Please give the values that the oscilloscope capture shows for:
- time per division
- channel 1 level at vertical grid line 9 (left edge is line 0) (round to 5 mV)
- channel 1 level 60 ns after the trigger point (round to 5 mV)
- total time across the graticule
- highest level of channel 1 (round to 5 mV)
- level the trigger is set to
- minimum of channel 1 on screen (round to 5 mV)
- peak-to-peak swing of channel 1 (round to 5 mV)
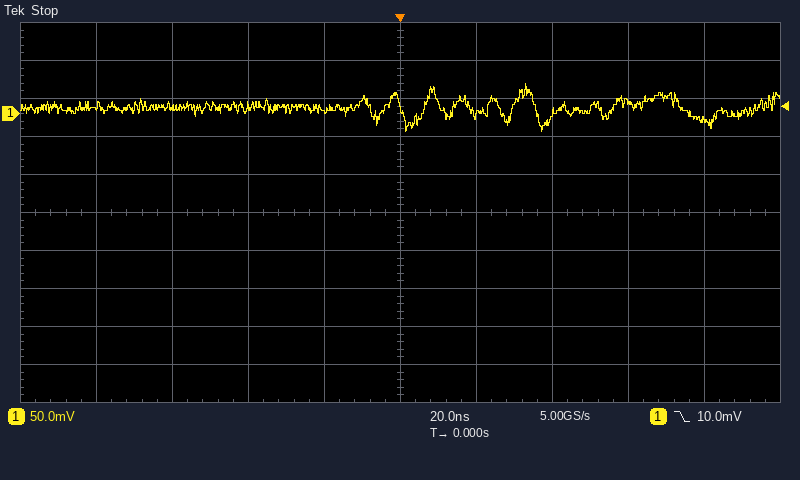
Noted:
20 ns
-10 mV
15 mV
200 ns
40 mV
10.0 mV
-25 mV
65 mV
